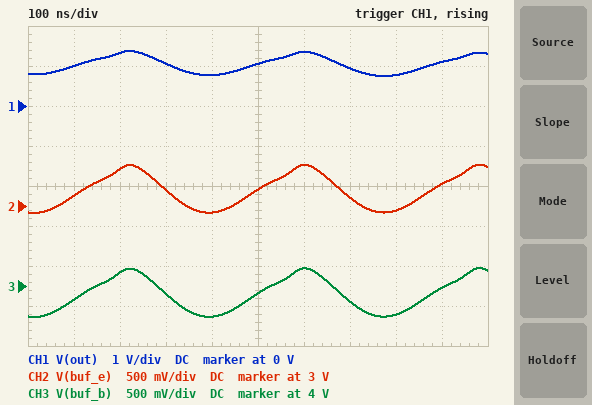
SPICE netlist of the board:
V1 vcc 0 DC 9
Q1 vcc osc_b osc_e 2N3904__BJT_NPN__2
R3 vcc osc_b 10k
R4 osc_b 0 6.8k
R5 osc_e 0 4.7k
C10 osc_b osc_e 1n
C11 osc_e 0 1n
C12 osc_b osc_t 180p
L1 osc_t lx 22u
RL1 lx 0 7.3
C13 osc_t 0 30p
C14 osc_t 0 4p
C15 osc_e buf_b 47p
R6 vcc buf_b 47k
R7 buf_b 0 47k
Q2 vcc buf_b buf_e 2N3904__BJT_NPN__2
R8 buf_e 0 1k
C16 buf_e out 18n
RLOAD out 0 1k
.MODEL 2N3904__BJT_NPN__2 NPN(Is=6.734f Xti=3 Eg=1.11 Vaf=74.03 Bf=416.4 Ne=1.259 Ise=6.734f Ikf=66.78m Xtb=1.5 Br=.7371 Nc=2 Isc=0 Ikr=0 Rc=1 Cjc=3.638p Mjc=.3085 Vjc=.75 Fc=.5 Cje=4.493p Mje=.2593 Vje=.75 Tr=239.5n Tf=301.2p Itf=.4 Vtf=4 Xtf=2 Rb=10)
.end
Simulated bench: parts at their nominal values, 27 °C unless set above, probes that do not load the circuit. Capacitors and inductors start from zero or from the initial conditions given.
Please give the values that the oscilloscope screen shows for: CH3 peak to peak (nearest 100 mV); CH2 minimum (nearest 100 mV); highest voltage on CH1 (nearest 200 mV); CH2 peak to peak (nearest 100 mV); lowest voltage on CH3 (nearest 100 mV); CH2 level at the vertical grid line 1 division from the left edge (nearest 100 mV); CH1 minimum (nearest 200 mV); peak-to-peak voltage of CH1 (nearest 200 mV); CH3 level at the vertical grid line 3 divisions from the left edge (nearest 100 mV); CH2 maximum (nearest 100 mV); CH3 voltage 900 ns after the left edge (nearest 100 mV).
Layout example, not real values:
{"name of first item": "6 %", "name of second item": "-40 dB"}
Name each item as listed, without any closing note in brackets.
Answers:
{"CH3 peak to peak": "600 mV", "CH2 minimum": "2.9 V", "highest voltage on CH1": "1.4 V", "CH2 peak to peak": "600 mV", "lowest voltage on CH3": "3.6 V", "CH2 level at the vertical grid line 1 division from the left edge": "3.1 V", "CH1 minimum": "800 mV", "peak-to-peak voltage of CH1": "600 mV", "CH3 level at the vertical grid line 3 divisions from the left edge": "3.9 V", "CH2 maximum": "3.5 V", "CH3 voltage 900 ns after the left edge": "4.0 V"}
